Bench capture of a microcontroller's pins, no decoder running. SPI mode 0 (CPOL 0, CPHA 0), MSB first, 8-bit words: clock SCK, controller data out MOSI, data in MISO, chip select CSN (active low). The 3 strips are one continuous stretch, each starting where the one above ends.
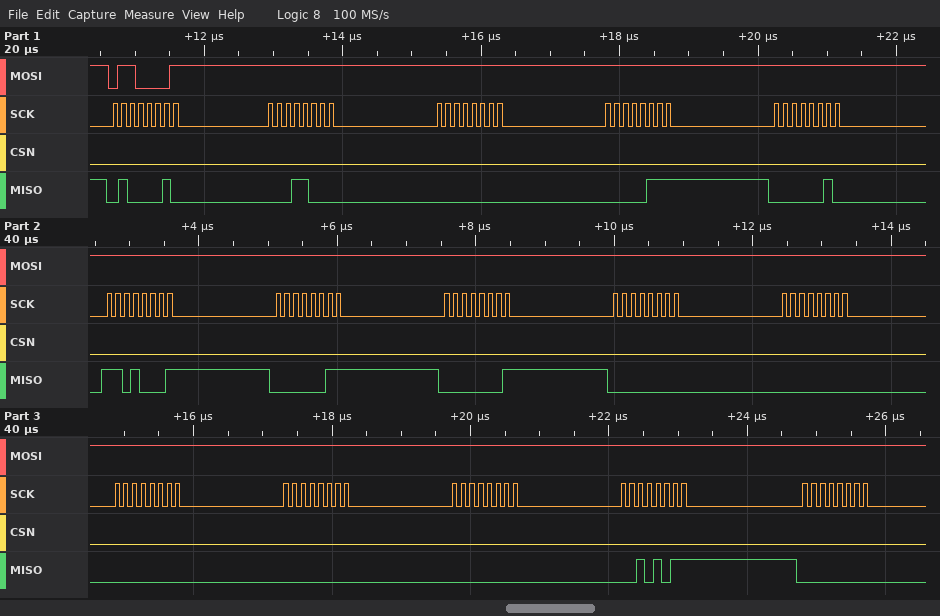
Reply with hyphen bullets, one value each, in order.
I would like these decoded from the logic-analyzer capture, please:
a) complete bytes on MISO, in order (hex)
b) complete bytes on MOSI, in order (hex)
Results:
- 42 18 00 07 02 D1 03 01 00 00 00 00 00 2B 00
- 61 FF FF FF FF FF FF FF FF FF FF FF FF FF FF
